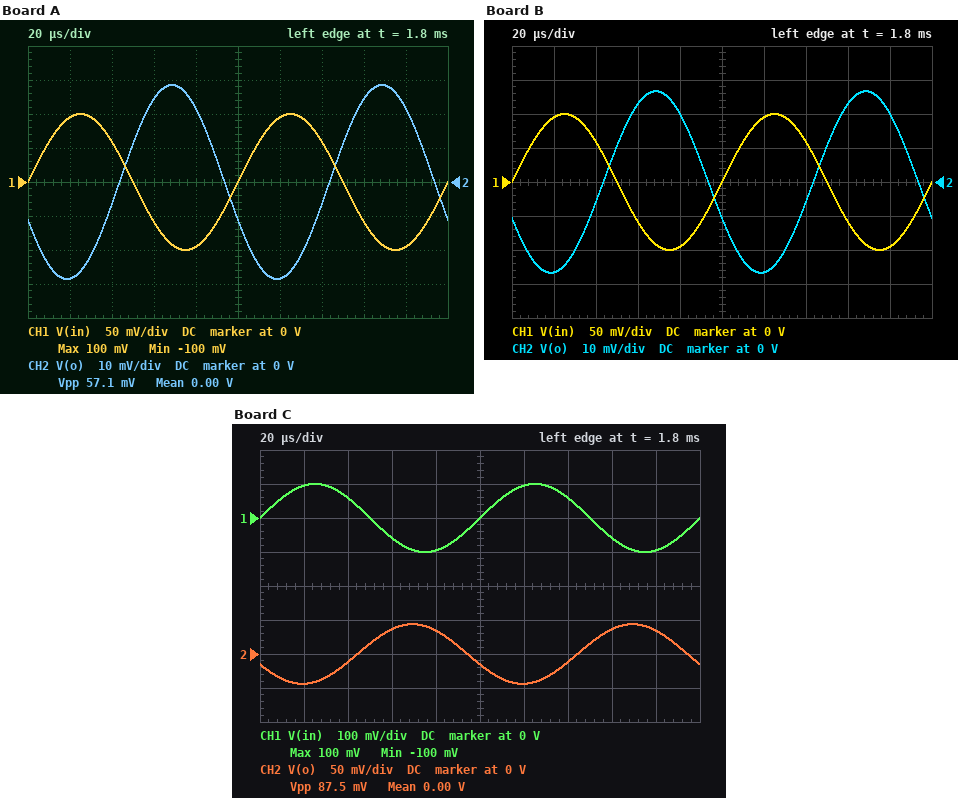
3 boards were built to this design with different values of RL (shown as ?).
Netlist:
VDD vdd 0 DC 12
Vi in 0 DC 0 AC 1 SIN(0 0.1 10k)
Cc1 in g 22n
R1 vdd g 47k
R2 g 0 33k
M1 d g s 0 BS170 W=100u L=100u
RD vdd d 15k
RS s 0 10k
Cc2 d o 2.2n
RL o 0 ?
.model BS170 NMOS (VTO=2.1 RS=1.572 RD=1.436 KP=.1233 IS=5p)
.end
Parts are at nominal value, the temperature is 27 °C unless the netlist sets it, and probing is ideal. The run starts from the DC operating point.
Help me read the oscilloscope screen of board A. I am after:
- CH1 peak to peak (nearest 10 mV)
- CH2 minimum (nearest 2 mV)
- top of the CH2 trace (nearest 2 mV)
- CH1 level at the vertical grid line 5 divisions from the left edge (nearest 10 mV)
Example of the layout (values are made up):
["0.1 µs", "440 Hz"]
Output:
["200 mV", "-28 mV", "28 mV", "0 V"]
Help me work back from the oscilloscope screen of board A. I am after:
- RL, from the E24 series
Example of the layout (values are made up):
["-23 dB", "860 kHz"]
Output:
["3.9 kΩ"]
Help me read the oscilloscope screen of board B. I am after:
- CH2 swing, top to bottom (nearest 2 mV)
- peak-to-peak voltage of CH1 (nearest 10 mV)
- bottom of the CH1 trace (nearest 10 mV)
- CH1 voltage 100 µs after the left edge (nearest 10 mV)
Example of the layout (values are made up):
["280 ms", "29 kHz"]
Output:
["54 mV", "200 mV", "-100 mV", "0 V"]
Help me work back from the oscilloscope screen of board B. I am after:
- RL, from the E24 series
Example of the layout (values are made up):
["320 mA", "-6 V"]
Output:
["3.6 kΩ"]
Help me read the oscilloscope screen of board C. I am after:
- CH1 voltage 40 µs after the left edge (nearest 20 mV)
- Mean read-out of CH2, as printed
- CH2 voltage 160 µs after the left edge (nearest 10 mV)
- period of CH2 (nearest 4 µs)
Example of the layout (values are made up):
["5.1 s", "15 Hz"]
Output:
["60 mV", "0.00 V", "40 mV", "100 µs"]
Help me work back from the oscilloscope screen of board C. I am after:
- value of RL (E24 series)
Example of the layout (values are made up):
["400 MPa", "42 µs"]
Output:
["6.8 kΩ"]
